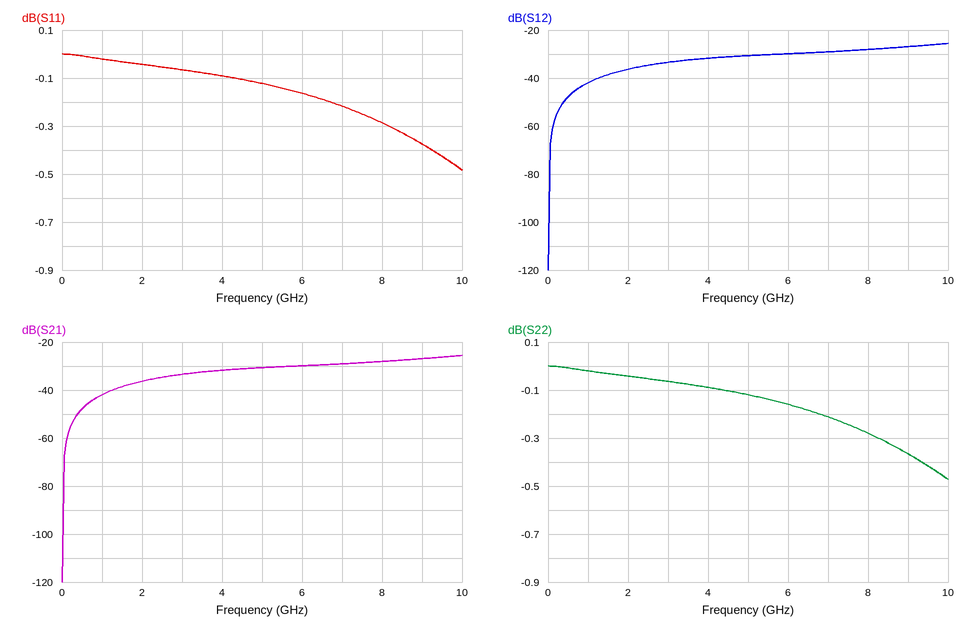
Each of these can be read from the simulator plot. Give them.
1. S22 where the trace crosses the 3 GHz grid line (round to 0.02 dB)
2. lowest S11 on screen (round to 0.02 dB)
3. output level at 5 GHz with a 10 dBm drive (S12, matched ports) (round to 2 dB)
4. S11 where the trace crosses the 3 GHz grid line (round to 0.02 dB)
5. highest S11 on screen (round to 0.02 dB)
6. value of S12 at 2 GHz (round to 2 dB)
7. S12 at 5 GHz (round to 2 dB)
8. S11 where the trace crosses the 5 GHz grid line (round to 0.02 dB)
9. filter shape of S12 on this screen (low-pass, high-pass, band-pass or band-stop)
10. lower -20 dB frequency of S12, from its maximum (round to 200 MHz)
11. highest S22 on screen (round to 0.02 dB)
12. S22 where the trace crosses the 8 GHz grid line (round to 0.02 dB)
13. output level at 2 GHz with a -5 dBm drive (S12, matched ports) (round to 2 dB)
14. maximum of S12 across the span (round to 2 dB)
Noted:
-0.06 dB
-0.48 dB
-20 dBm
-0.06 dB
0.00 dB
-36 dB
-30 dB
-0.12 dB
high-pass
600 MHz
0.00 dB
-0.28 dB
-42 dBm
-26 dB
